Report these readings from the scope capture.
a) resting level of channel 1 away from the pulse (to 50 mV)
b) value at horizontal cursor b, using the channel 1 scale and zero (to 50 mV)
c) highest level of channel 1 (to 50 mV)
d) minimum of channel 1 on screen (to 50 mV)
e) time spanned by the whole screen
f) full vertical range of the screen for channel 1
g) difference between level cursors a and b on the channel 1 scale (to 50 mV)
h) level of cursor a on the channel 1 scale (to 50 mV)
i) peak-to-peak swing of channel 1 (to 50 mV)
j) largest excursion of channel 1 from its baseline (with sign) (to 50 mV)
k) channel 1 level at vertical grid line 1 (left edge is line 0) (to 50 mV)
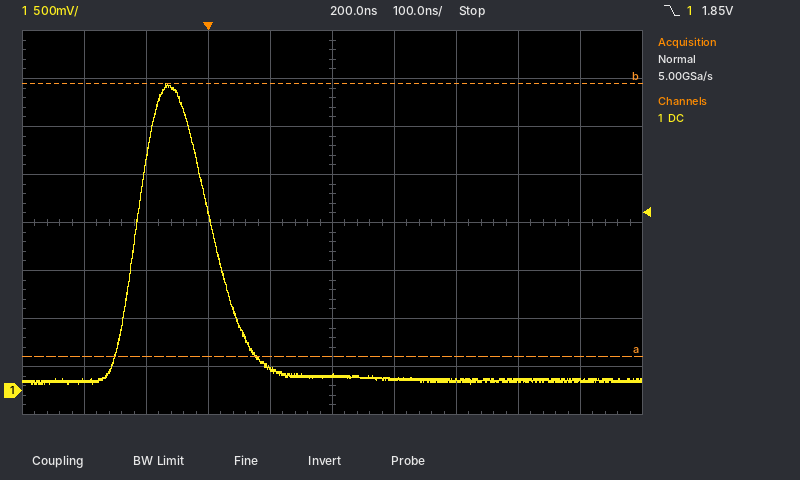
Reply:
100 mV
3.20 V
3.20 V
50 mV
1 µs
4 V
2.85 V
350 mV
3.15 V
+3.10 V
100 mV
